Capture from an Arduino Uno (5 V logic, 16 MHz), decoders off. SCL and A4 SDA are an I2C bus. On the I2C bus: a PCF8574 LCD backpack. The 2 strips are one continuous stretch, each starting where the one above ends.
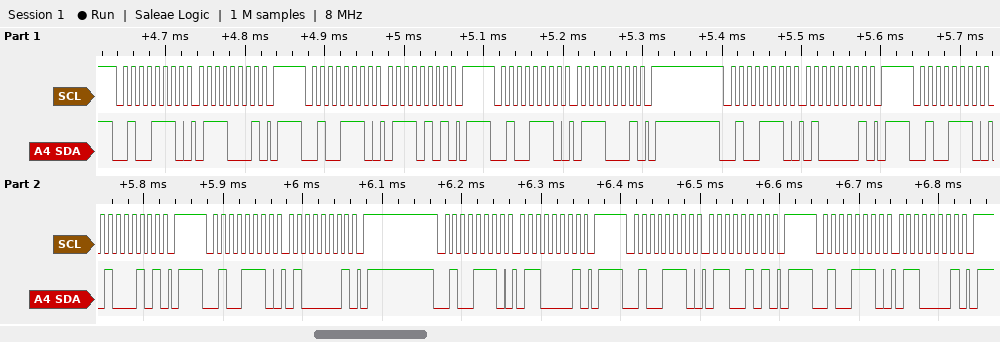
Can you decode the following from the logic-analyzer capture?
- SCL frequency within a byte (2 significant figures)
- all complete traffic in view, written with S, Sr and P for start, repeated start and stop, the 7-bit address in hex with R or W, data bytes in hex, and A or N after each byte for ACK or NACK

100 kHz
S 27W A 71 A P S 27W A 75 A P S 27W A 71 A P S 27W A 41 A P S 27W A 45 A P S 27W A 41 A P S 27W A 61 A P S 27W A 65 A P S 27W A 61 A P
